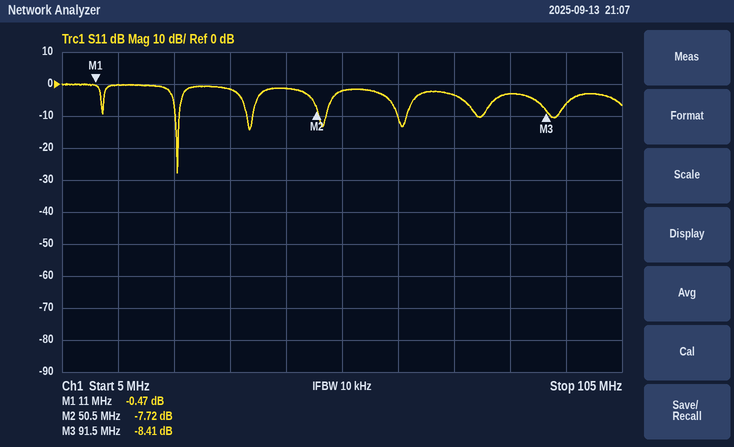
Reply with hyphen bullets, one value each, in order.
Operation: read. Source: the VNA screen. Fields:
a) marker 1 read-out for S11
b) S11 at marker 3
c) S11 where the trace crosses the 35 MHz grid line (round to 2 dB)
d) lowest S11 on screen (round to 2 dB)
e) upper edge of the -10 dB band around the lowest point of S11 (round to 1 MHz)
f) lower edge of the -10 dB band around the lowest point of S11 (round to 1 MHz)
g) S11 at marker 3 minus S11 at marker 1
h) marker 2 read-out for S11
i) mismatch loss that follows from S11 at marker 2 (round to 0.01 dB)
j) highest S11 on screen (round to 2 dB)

- -0.47 dB
- -8.41 dB
- -2 dB
- -28 dB
- 26 MHz
- 25 MHz
- -7.94 dB
- -7.72 dB
- 0.80 dB
- 0 dB
